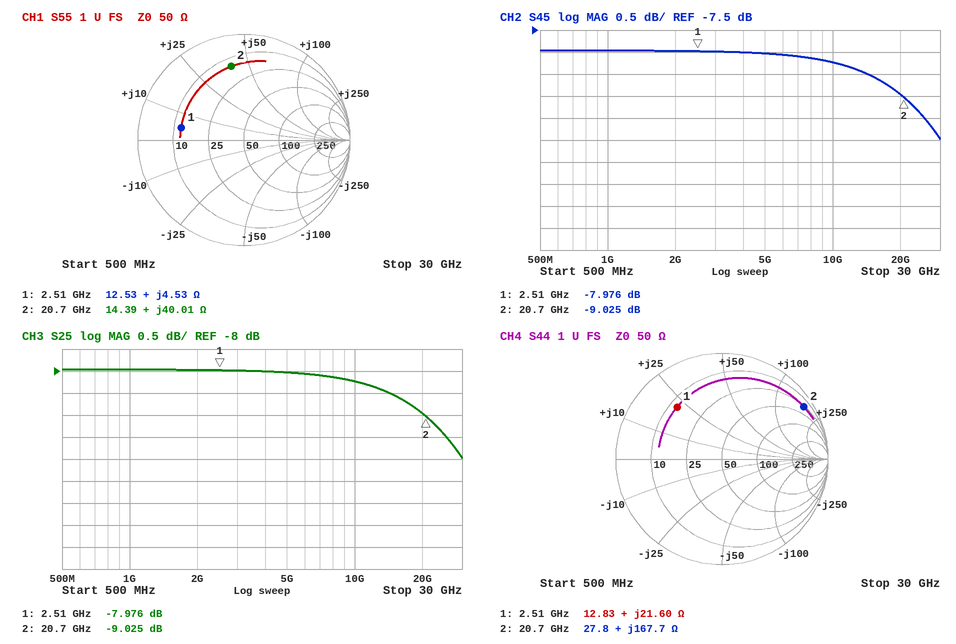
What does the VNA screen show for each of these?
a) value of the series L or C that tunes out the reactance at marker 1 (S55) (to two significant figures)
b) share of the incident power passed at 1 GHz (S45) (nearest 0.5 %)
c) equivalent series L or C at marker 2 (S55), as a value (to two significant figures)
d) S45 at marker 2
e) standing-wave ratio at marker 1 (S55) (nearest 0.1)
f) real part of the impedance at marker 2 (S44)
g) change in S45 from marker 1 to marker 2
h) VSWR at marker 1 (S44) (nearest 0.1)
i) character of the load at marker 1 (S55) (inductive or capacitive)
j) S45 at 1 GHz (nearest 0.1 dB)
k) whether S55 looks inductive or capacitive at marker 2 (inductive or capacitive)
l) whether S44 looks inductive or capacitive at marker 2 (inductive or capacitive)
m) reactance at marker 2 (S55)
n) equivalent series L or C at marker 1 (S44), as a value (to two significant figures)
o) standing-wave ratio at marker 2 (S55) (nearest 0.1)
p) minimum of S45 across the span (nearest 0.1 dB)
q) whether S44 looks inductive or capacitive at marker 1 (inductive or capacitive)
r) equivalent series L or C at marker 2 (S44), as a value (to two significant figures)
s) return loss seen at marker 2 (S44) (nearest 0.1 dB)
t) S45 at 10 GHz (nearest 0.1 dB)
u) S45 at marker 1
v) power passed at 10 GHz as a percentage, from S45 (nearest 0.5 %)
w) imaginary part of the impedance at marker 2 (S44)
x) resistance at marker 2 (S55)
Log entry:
14 pF
16.0 %
310 pH
-9.025 dB
4.0
27.8 Ω
-1.049 dB
4.7
inductive
-8.0 dB
inductive
inductive
+40.01 Ω
1.4 nH
5.8
-10.0 dB
inductive
1.3 nH
0.8 dB
-8.2 dB
-7.976 dB
15.0 %
+167.7 Ω
14.39 Ω
